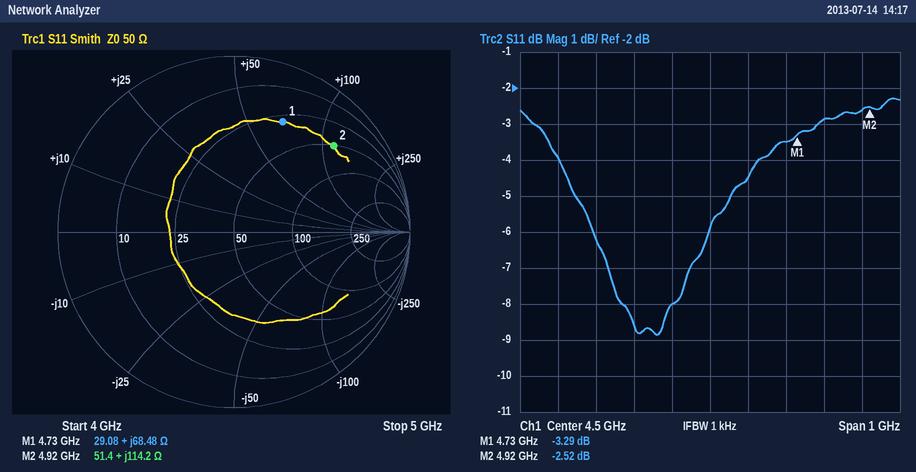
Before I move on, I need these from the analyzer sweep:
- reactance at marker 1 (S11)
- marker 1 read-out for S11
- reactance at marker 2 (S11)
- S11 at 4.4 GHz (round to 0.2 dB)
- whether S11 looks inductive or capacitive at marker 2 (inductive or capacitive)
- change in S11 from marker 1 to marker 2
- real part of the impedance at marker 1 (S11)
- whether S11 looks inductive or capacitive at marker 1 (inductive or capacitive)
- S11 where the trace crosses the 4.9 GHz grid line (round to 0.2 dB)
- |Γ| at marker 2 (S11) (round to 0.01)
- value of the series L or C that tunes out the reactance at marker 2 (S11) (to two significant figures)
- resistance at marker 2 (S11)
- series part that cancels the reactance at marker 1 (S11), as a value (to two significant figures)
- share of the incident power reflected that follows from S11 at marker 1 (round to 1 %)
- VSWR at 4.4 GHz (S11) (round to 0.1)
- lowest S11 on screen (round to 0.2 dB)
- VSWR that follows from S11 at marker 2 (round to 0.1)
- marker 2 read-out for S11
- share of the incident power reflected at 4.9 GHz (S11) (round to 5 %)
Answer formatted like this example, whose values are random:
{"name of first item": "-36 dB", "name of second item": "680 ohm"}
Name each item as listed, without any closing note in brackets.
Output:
{"reactance at marker 1": "+68.48 Ω", "marker 1 read-out for S11": "-3.29 dB", "reactance at marker 2": "+114.2 Ω", "S11 at 4.4 GHz": "-8.0 dB", "whether S11 looks inductive or capacitive at marker 2": "inductive", "change in S11 from marker 1 to marker 2": "0.77 dB", "real part of the impedance at marker 1": "29.08 Ω", "whether S11 looks inductive or capacitive at marker 1": "inductive", "S11 where the trace crosses the 4.9 GHz grid line": "-2.6 dB", "|Γ| at marker 2 (S11)": "0.75", "value of the series L or C that tunes out the reactance at marker 2 (S11)": "280 fF", "resistance at marker 2": "51.4 Ω", "series part that cancels the reactance at marker 1 (S11), as a value": "490 fF", "share of the incident power reflected that follows from S11 at marker 1": "47 %", "VSWR at 4.4 GHz (S11)": "2.3", "lowest S11 on screen": "-8.8 dB", "VSWR that follows from S11 at marker 2": "6.9", "marker 2 read-out for S11": "-2.52 dB", "share of the incident power reflected at 4.9 GHz (S11)": "55 %"}
